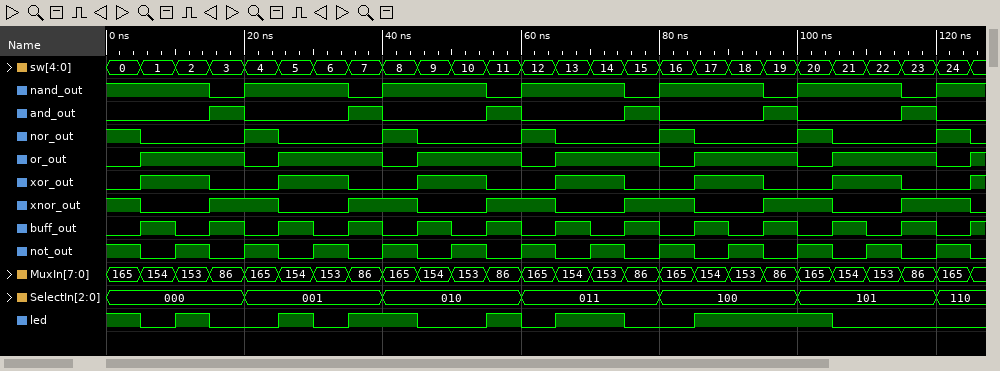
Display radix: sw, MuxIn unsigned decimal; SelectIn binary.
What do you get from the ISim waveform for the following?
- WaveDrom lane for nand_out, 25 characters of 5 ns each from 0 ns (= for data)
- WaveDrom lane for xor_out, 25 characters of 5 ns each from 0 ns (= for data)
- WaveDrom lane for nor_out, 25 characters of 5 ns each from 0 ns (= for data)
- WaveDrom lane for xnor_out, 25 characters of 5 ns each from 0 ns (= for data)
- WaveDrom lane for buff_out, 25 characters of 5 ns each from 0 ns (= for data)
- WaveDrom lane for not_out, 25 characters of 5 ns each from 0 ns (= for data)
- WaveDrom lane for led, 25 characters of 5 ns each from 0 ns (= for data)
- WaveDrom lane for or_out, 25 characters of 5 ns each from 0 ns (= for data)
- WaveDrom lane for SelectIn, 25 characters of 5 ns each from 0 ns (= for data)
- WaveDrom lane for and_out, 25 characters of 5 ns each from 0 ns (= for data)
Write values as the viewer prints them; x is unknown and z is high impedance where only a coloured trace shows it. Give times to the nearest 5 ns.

{name: 'nand_out', wave: '1..01..01..01..01..01..01'}
{name: 'xor_out', wave: '01.0.1.0.1.0.1.0.1.0.1.0.'}
{name: 'nor_out', wave: '10..10..10..10..10..10..1'}
{name: 'xnor_out', wave: '10.1.0.1.0.1.0.1.0.1.0.1.'}
{name: 'buff_out', wave: '0101010101010101010101010'}
{name: 'not_out', wave: '1010101010101010101010101'}
{name: 'led', wave: '1010.101.0.101.0.1...0...'}
{name: 'or_out', wave: '01..01..01..01..01..01..0'}
{name: 'SelectIn', wave: '=...=...=...=...=...=...=', data: '000 001 010 011 100 101 110'}
{name: 'and_out', wave: '0..10..10..10..10..10..10'}
